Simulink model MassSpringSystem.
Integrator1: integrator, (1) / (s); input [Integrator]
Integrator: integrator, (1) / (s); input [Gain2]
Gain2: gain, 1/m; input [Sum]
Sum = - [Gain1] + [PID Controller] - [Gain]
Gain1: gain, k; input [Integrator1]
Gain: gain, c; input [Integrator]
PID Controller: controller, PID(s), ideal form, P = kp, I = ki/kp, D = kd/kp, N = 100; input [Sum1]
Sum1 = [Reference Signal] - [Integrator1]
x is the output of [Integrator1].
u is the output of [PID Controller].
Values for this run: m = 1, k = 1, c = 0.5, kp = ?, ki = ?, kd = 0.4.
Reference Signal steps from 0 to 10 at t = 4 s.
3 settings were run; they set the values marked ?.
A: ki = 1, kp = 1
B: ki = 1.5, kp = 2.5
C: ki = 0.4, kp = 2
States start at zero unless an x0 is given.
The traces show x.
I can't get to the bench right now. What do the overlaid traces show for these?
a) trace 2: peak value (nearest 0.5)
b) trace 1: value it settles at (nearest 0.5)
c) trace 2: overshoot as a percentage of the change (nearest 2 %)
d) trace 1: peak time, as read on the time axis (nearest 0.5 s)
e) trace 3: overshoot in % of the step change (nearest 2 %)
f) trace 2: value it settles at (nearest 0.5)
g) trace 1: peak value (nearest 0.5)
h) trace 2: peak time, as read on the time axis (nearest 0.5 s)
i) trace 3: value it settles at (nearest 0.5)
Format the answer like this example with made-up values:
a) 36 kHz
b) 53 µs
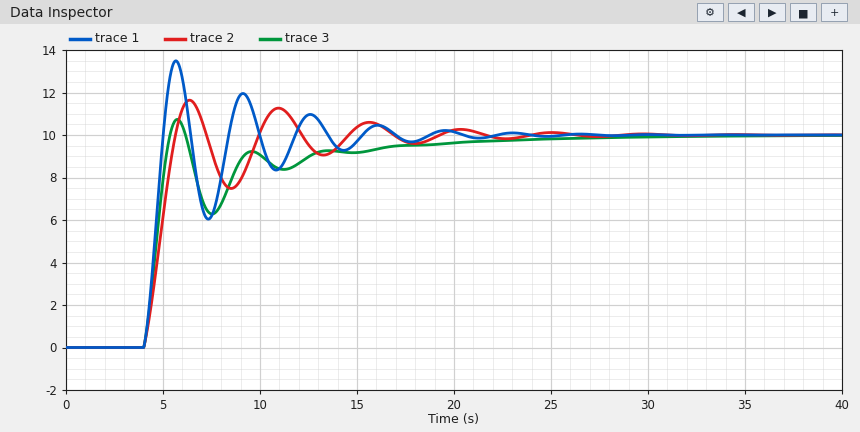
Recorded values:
a) 11.5
b) 10.0
c) 16 %
d) 5.5 s
e) 8 %
f) 10.0
g) 13.5
h) 6.5 s
i) 10.0
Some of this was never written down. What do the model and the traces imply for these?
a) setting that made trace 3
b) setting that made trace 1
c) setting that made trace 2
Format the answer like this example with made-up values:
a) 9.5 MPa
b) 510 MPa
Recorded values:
a) C
b) B
c) A
